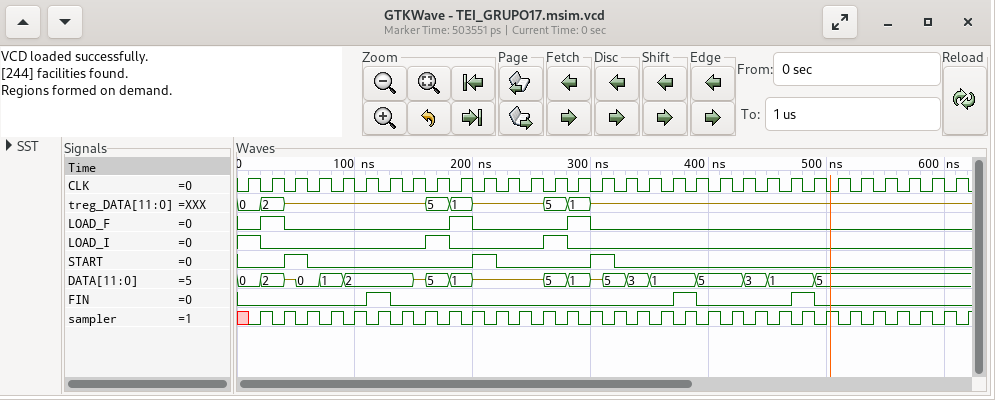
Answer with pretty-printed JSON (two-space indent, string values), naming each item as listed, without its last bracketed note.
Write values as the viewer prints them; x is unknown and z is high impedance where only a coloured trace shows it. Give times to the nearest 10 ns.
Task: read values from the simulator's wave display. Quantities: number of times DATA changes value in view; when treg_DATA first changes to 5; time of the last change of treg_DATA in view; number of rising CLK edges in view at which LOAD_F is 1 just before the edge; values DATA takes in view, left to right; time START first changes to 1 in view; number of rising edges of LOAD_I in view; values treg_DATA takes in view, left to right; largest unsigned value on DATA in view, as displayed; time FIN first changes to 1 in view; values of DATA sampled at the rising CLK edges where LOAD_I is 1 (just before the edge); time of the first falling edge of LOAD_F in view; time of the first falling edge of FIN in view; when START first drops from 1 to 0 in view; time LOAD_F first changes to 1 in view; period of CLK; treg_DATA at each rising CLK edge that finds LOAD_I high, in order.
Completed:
{
  "number of times DATA changes value in view": "19",
  "when treg_DATA first changes to 5": "160 ns",
  "time of the last change of treg_DATA in view": "300 ns",
  "number of rising CLK edges in view at which LOAD_F is 1 just before the edge": "3",
  "values DATA takes in view, left to right": "0, 2, z, 0, 1, 2, z, 5, 1, z, 5, 1, z, 5, 3, 1, 5, 3, 1, 5",
  "time START first changes to 1 in view": "40 ns",
  "number of rising edges of LOAD_I in view": "2",
  "values treg_DATA takes in view, left to right": "0, 2, z, 5, 1, z, 5, 1, z",
  "largest unsigned value on DATA in view, as displayed": "5",
  "time FIN first changes to 1 in view": "110 ns",
  "values of DATA sampled at the rising CLK edges where LOAD_I is 1": "0, 5, 5",
  "time of the first falling edge of LOAD_F in view": "40 ns",
  "time of the first falling edge of FIN in view": "130 ns",
  "when START first drops from 1 to 0 in view": "60 ns",
  "time LOAD_F first changes to 1 in view": "20 ns",
  "period of CLK": "20 ns",
  "treg_DATA at each rising CLK edge that finds LOAD_I high, in order": "0, 5, 5"
}
